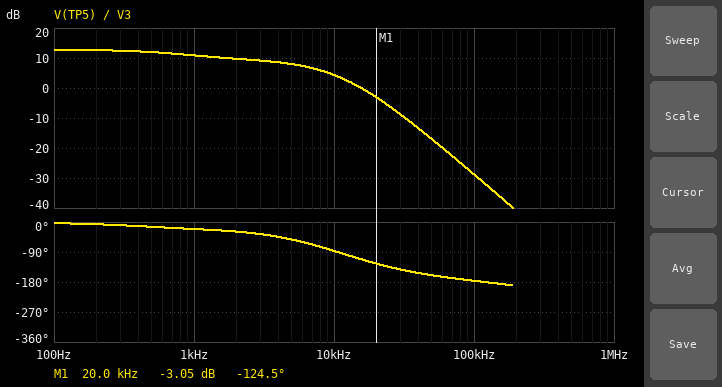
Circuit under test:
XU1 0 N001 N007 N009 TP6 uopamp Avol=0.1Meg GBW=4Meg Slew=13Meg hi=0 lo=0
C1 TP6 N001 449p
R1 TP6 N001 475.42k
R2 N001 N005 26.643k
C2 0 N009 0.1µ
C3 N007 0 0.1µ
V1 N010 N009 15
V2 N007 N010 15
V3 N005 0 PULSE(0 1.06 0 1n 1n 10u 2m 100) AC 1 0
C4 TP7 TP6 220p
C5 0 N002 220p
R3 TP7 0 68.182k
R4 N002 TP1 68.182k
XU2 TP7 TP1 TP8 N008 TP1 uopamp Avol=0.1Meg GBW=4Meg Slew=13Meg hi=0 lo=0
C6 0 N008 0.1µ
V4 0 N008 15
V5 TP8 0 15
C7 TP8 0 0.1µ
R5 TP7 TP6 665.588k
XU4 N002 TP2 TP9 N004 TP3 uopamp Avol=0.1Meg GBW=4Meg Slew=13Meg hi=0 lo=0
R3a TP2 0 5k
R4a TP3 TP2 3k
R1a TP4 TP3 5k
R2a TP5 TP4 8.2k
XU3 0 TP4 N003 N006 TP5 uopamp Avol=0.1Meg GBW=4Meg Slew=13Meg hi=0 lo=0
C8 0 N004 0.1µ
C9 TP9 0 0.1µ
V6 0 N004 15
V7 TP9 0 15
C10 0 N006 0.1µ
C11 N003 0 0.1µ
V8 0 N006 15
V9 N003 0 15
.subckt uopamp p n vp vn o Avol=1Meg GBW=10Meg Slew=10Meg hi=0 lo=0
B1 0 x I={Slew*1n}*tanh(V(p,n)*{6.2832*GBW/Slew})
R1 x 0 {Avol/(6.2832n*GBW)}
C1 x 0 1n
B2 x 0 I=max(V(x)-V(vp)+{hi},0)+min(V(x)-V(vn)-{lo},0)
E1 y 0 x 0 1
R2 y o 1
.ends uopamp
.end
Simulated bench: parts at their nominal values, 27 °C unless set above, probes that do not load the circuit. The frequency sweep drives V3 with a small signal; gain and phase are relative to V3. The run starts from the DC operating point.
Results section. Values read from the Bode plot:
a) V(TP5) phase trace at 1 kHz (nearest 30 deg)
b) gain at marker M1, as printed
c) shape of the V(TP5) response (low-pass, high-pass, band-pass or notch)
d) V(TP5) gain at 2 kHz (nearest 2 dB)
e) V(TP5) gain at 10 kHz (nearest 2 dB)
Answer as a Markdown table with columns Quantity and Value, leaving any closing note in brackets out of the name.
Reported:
| Quantity | Value |
|---|---|
| V(TP5) phase trace at 1 kHz | -30 deg |
| gain at marker M1, as printed | -3.05 dB |
| shape of the V(TP5) response | low-pass |
| V(TP5) gain at 2 kHz | 10 dB |
| V(TP5) gain at 10 kHz | 4 dB |
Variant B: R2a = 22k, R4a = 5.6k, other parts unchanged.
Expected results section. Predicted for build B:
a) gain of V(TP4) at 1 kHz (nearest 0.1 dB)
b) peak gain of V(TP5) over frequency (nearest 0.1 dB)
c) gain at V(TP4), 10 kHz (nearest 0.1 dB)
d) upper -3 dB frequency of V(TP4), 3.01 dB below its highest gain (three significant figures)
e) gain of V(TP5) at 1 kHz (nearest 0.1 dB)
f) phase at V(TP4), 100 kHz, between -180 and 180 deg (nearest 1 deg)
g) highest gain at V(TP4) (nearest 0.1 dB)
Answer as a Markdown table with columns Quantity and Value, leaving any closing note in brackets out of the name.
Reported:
| Quantity | Value |
|---|---|
| gain of V(TP4) at 1 kHz | -50.1 dB |
| peak gain of V(TP5) over frequency | 23.8 dB |
| gain at V(TP4), 10 kHz | -36.7 dB |
| upper -3 dB frequency of V(TP4), 3.01 dB below its highest gain | 26.8 kHz |
| gain of V(TP5) at 1 kHz | 21.9 dB |
| phase at V(TP4), 100 kHz, between -180 and 180 deg | 89 deg |
| highest gain at V(TP4) | -36.6 dB |
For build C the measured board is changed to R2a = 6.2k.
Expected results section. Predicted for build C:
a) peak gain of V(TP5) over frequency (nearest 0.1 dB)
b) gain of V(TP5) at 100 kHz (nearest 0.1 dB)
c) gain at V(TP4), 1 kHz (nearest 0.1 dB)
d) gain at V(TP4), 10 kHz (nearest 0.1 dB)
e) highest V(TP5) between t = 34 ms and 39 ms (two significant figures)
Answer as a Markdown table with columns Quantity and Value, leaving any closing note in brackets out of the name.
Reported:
| Quantity | Value |
|---|---|
| peak gain of V(TP5) over frequency | 10.3 dB |
| gain of V(TP5) at 100 kHz | -31.2 dB |
| gain at V(TP4), 1 kHz | -63.6 dB |
| gain at V(TP4), 10 kHz | -50.1 dB |
| highest V(TP5) between t = 34 ms and 39 ms | 6.7 mV |
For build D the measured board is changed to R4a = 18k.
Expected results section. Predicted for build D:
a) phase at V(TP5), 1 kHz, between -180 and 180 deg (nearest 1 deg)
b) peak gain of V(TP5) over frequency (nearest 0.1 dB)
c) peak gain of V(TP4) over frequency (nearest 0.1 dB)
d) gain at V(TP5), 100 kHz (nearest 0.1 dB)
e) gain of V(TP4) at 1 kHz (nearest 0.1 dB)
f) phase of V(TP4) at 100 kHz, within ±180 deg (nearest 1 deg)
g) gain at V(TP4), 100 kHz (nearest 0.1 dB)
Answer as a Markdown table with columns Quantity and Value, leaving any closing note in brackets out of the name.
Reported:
| Quantity | Value |
|---|---|
| phase at V(TP5), 1 kHz, between -180 and 180 deg | -21 deg |
| peak gain of V(TP5) over frequency | 21.9 dB |
| peak gain of V(TP4) over frequency | -38.5 dB |
| gain at V(TP5), 100 kHz | -19.7 dB |
| gain of V(TP4) at 1 kHz | -52.0 dB |
| phase of V(TP4) at 100 kHz, within ±180 deg | 89 deg |
| gain at V(TP4), 100 kHz | -51.7 dB |
